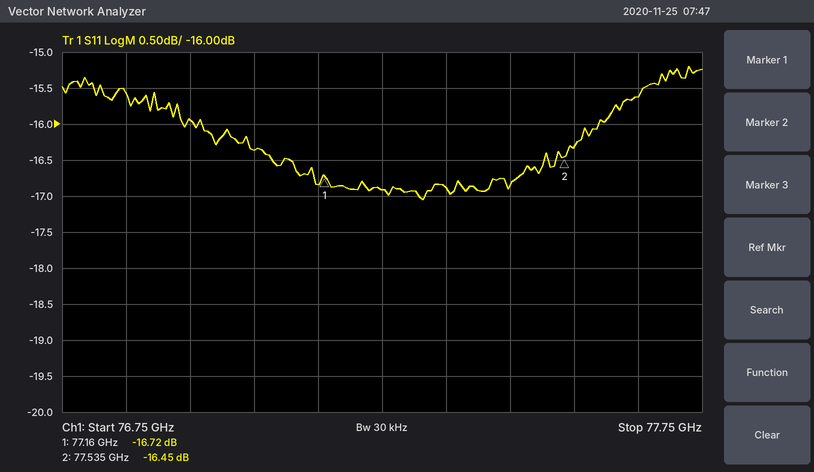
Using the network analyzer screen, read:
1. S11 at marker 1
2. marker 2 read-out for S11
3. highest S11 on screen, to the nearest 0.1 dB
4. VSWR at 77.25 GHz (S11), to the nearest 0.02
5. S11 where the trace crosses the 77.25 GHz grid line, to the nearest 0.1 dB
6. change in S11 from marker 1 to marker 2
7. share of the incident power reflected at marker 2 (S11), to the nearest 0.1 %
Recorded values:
-16.72 dB
-16.45 dB
-15.2 dB
1.34
-16.9 dB
0.27 dB
2.3 %
